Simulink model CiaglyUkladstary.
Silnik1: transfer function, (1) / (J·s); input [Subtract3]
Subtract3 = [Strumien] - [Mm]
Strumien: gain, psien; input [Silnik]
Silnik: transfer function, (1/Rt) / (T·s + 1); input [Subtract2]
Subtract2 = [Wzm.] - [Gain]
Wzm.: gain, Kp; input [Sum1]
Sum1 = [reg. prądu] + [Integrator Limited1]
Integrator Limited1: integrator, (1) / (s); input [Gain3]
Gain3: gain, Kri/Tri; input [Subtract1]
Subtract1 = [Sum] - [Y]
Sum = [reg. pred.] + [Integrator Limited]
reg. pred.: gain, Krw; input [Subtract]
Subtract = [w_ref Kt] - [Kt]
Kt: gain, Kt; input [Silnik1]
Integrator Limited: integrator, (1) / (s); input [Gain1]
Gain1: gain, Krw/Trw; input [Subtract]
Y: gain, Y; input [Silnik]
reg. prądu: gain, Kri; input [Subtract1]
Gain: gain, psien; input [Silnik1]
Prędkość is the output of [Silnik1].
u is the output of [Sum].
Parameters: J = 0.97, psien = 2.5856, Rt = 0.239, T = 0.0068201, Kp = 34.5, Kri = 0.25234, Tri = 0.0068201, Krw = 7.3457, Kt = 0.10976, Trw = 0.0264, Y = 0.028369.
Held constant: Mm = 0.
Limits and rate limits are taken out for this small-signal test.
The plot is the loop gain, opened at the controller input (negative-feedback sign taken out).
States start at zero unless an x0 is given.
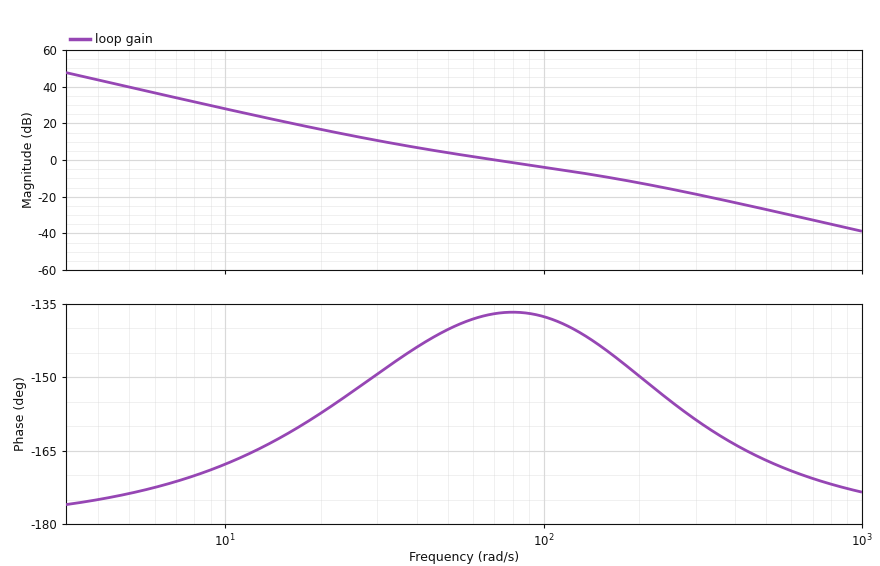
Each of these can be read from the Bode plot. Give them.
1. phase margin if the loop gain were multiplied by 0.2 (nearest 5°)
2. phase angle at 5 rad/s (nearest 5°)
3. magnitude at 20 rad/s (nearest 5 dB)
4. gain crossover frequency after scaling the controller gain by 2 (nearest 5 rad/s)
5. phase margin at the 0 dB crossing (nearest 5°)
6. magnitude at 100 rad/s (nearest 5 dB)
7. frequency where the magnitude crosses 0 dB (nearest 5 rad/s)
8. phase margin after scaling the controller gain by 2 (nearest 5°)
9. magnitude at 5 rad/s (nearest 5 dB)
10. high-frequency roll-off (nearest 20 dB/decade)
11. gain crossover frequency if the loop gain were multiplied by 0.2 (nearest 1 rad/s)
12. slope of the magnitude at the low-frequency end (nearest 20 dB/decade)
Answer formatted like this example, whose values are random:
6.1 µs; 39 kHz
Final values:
25°; -175°; 15 dB; 120 rad/s; 45°; -5 dB; 70 rad/s; 40°; 40 dB; -40 dB/decade; 24 rad/s; -40 dB/decade
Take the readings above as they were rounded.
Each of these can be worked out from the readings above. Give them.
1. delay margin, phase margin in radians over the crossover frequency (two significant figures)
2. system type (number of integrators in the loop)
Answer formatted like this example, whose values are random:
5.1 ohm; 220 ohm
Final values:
0.011 s; 2
